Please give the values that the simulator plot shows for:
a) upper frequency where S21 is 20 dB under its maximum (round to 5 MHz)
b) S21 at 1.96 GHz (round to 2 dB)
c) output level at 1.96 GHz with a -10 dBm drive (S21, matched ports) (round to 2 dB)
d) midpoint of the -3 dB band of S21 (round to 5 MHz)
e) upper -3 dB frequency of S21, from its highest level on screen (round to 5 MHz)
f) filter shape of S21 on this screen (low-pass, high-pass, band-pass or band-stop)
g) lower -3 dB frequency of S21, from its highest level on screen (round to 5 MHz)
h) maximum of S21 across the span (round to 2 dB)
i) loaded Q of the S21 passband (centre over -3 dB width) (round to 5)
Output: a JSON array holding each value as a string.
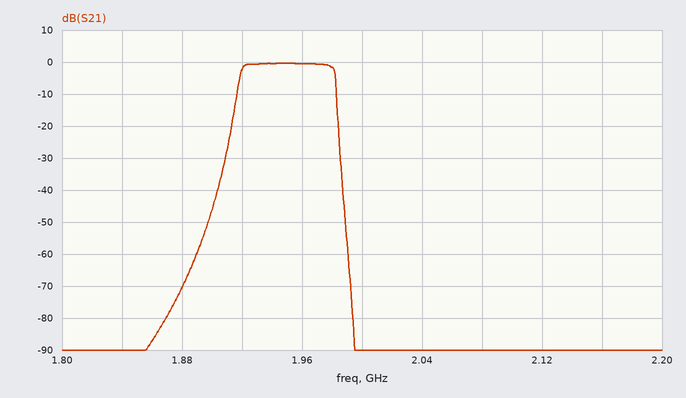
["1.985 GHz", "0 dB", "-10 dBm", "1.950 GHz", "1.980 GHz", "band-pass", "1.920 GHz", "0 dB", "30"]
